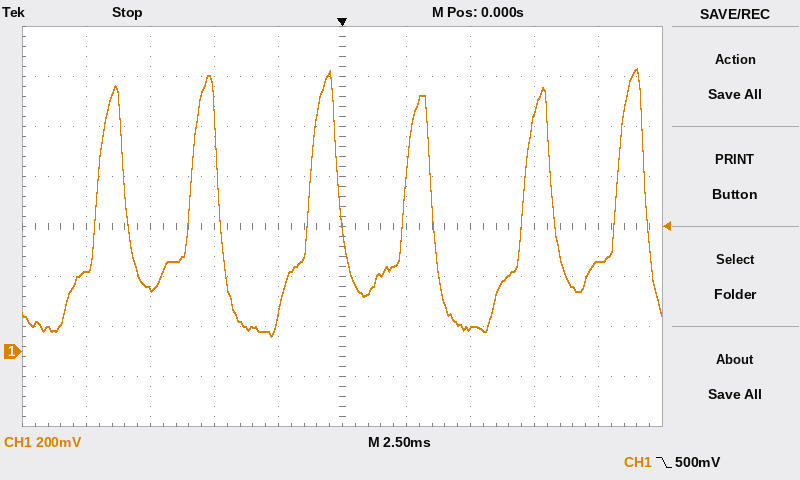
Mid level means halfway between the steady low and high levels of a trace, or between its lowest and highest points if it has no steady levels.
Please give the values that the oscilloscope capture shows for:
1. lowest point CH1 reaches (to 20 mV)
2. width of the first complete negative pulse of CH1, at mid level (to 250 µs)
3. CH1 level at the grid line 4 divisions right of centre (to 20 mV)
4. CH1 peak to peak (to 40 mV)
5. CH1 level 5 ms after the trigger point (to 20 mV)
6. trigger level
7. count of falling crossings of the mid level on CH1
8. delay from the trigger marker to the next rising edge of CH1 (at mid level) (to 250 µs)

60 mV
2.50 ms
360 mV
1.08 V
100 mV
500 mV
6
2.50 ms
